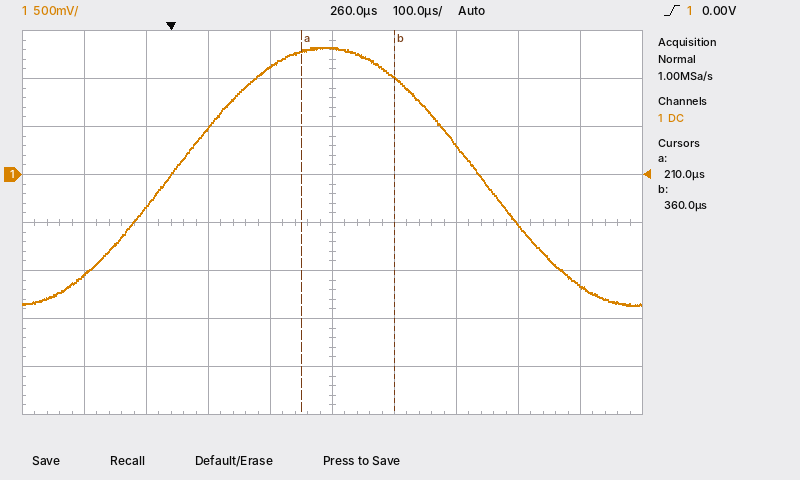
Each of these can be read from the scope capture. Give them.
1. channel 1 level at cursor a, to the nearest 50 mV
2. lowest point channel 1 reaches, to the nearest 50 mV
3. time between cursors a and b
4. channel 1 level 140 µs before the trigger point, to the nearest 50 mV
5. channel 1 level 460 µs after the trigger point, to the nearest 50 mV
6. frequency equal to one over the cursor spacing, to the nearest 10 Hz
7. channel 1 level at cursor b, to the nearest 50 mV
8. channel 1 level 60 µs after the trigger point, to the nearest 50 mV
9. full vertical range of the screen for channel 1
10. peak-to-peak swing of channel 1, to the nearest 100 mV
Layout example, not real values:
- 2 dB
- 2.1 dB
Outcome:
- 1.30 V
- -1.35 V
- 150 µs
- -1.05 V
- 300 mV
- 6.67 kHz
- 1.00 V
- 500 mV
- 4 V
- 2.70 V
